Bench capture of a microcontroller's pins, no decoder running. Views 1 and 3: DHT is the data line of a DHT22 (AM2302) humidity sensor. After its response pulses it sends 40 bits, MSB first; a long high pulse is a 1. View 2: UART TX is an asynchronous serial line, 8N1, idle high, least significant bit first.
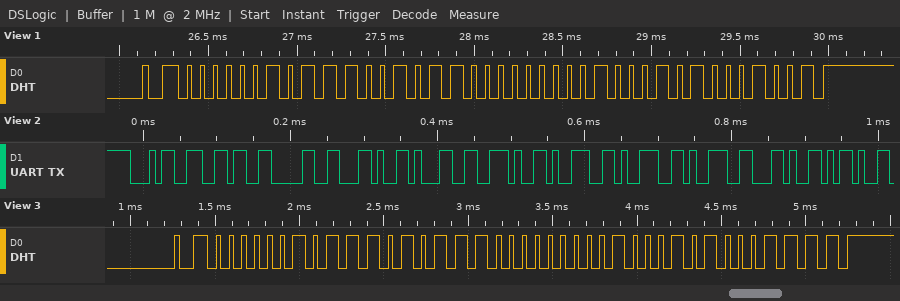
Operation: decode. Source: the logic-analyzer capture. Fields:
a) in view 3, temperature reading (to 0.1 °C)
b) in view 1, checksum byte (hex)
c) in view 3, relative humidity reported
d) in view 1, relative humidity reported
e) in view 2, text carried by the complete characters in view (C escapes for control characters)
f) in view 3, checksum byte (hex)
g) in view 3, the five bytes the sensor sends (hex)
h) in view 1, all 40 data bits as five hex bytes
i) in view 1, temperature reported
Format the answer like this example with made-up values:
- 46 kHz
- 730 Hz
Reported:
- -3.4 °C
- 0x89
- 74.7 %
- 74.1 %
- "460,1.999,-"
- 0x8F
- 02 EB 80 22 8F
- 02 E5 80 22 89
- -3.4 °C
